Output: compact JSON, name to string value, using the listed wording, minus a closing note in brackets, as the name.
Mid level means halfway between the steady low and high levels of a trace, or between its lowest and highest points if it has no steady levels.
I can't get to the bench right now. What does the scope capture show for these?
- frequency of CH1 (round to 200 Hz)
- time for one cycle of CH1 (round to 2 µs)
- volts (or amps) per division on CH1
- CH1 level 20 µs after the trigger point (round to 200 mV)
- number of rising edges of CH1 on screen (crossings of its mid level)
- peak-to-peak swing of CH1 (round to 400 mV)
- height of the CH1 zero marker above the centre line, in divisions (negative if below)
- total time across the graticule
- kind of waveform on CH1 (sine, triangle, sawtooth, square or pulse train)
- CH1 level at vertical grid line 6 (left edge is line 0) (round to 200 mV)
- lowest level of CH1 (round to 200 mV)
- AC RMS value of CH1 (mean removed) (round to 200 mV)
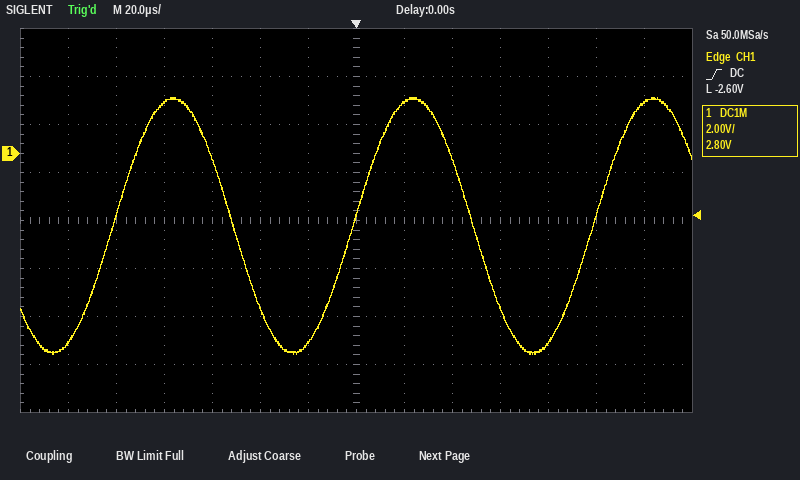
{"frequency of CH1": "10.0 kHz", "time for one cycle of CH1": "100 µs", "volts (or amps) per division on CH1": "2 V", "CH1 level 20 µs after the trigger point": "2.2 V", "number of rising edges of CH1 on screen": "3", "peak-to-peak swing of CH1": "10.8 V", "height of the CH1 zero marker above the centre line, in divisions": "+1.4 div", "total time across the graticule": "280 µs", "kind of waveform on CH1": "sine", "CH1 level at vertical grid line 6 (left edge is line 0)": "-7.8 V", "lowest level of CH1": "-8.4 V", "AC RMS value of CH1 (mean removed)": "3.8 V"}
